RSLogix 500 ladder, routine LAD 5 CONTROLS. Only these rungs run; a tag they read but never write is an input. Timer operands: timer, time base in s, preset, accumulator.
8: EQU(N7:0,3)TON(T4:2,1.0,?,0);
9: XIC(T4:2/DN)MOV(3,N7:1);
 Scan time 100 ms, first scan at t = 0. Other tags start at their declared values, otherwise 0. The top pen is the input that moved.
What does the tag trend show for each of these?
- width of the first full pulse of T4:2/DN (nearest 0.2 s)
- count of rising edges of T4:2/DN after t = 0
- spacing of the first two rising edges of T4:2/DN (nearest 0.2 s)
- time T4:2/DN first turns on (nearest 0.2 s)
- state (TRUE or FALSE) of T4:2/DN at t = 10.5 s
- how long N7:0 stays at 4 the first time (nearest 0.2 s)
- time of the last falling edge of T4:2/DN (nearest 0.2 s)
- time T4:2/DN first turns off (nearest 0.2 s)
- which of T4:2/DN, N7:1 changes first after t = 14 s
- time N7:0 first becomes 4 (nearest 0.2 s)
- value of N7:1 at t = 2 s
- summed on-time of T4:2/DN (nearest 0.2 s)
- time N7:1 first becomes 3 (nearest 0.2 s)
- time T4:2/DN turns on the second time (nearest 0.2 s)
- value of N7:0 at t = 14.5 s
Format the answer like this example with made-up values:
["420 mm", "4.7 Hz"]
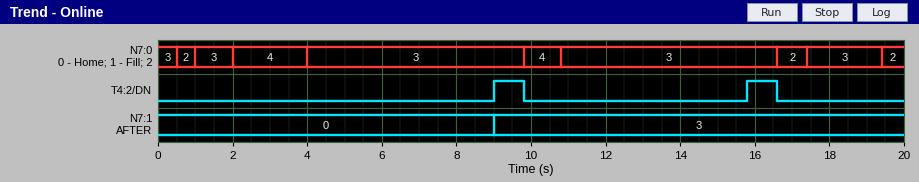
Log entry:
["0.8 s", "2", "6.8 s", "9.0 s", "FALSE", "2.0 s", "16.6 s", "9.8 s", "T4:2/DN", "2.0 s", "0", "1.6 s", "9.0 s", "15.8 s", "3"]
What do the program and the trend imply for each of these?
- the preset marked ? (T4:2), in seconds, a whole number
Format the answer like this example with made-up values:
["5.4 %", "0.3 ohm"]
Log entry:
["5 s"]
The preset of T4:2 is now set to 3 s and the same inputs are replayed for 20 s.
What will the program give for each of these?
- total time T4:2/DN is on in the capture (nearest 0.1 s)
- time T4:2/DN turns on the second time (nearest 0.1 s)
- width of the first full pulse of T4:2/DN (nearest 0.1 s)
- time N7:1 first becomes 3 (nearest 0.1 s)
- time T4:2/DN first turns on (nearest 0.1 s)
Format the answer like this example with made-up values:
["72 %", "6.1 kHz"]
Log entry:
["5.6 s", "13.8 s", "2.8 s", "7.0 s", "7.0 s"]
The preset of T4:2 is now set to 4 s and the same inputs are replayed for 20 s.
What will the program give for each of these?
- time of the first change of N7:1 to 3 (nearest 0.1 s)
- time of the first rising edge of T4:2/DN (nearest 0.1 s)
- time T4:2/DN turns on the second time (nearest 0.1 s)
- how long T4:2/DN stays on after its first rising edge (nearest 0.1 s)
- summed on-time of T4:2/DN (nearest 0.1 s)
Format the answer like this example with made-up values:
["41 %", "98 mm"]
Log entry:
["8.0 s", "8.0 s", "14.8 s", "1.8 s", "3.6 s"]
